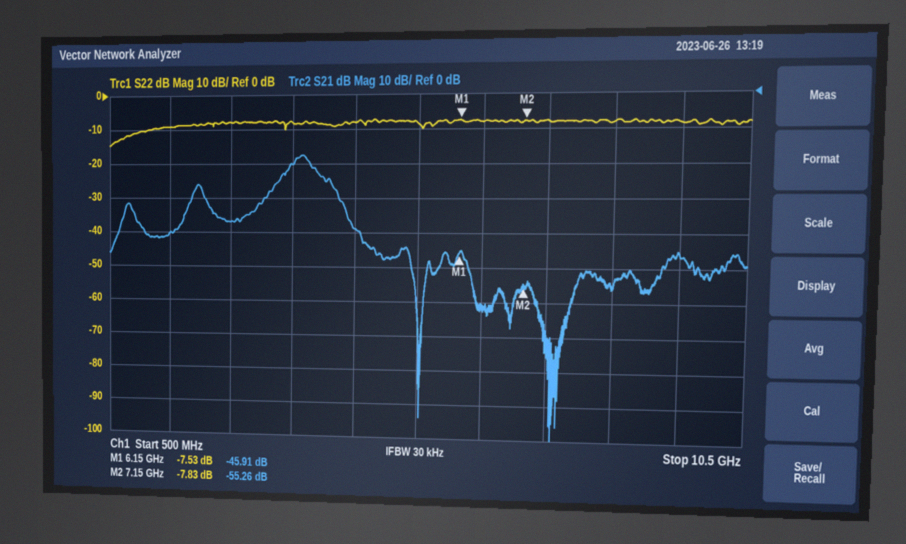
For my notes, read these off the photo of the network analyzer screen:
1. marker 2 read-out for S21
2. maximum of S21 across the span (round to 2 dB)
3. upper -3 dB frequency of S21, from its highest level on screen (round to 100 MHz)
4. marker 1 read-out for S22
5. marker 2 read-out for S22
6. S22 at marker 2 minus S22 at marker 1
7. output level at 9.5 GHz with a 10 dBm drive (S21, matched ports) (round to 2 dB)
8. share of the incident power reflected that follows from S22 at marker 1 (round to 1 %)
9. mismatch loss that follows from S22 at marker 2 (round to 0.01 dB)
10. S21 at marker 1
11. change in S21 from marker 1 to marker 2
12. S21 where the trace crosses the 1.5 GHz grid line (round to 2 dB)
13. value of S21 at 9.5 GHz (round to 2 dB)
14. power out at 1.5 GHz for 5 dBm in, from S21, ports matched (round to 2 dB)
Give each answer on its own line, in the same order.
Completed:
-55.26 dB
-18 dB
3.8 GHz
-7.53 dB
-7.83 dB
-0.30 dB
-36 dBm
18 %
0.78 dB
-45.91 dB
-9.35 dB
-40 dB
-46 dB
-36 dBm
